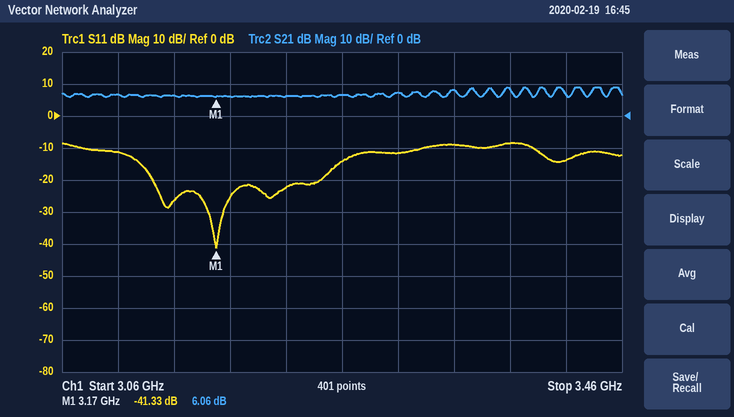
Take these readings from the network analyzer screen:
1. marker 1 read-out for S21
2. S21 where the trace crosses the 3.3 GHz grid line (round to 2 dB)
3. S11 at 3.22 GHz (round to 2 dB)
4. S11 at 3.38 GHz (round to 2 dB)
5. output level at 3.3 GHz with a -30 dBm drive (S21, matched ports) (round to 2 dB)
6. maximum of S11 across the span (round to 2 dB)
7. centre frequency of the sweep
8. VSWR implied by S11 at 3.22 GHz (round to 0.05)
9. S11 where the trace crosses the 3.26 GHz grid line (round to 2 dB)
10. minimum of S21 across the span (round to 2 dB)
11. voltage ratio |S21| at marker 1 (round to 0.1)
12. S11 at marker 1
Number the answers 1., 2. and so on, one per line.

1. 6.06 dB
2. 8 dB
3. -22 dB
4. -8 dB
5. -22 dBm
6. -8 dB
7. 3.26 GHz
8. 1.15
9. -14 dB
10. 6 dB
11. 2.0
12. -41.33 dB
